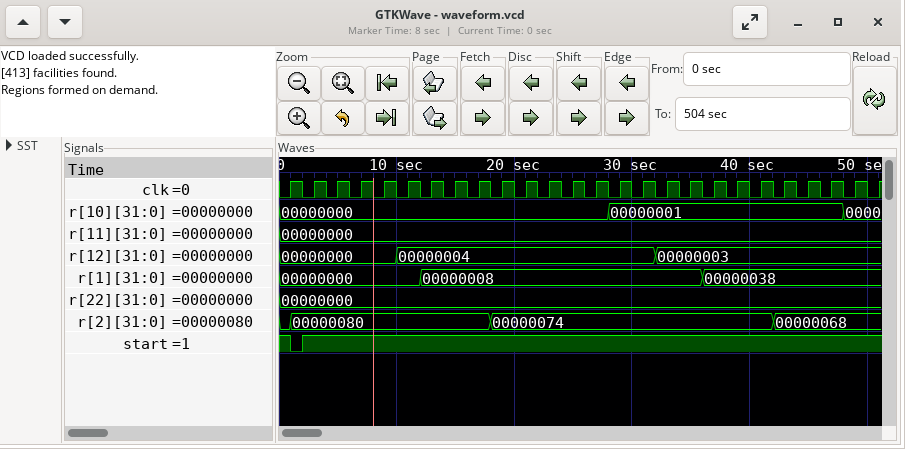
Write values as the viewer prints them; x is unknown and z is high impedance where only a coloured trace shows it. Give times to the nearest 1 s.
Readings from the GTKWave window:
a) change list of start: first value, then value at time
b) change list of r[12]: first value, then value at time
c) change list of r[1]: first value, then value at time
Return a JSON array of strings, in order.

["1, 0 at 1 s, 1 at 2 s", "00000000, 00000004 at 10 s, 00000003 at 32 s", "00000000, 00000008 at 12 s, 00000038 at 36 s"]
